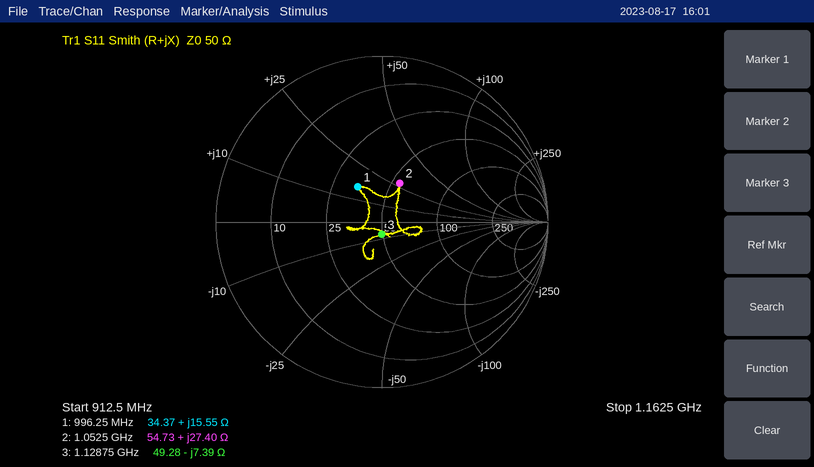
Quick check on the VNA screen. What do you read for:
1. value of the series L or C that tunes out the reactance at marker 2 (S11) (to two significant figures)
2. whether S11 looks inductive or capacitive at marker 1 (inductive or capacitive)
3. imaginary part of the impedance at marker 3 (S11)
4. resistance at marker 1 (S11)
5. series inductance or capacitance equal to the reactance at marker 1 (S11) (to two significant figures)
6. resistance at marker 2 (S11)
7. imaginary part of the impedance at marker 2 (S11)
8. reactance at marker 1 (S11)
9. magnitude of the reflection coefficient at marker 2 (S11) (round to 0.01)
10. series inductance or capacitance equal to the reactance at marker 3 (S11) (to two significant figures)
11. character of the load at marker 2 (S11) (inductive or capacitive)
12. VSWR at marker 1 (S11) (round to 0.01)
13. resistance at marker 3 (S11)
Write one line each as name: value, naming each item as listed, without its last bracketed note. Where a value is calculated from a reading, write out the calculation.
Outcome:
value of the series L or C that tunes out the reactance at marker 2 (S11): C = 1/(2π × 1.0525 GHz × 27.4 Ω) ≈ 5.5 pF
whether S11 looks inductive or capacitive at marker 1: inductive
imaginary part of the impedance at marker 3: -7.39 Ω
resistance at marker 1: 34.37 Ω
series inductance or capacitance equal to the reactance at marker 1 (S11): L = 15.55 Ω/(2π × 996.25 MHz) ≈ 2.5 nH
resistance at marker 2: 54.73 Ω
imaginary part of the impedance at marker 2: +27.40 Ω
reactance at marker 1: +15.55 Ω
magnitude of the reflection coefficient at marker 2 (S11): 0.26
series inductance or capacitance equal to the reactance at marker 3 (S11): C = 1/(2π × 1.12875 GHz × 7.39 Ω) ≈ 19 pF
character of the load at marker 2 (S11): inductive
VSWR at marker 1 (S11): 1.69
resistance at marker 3: 49.28 Ω
